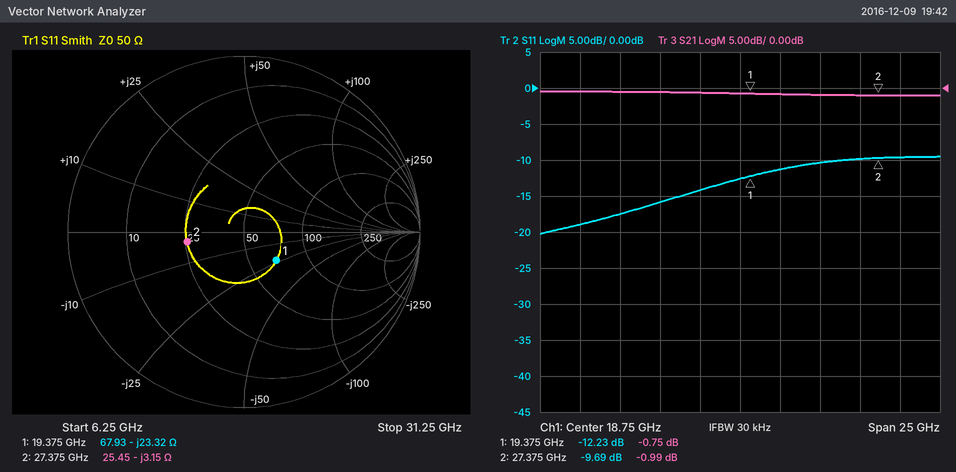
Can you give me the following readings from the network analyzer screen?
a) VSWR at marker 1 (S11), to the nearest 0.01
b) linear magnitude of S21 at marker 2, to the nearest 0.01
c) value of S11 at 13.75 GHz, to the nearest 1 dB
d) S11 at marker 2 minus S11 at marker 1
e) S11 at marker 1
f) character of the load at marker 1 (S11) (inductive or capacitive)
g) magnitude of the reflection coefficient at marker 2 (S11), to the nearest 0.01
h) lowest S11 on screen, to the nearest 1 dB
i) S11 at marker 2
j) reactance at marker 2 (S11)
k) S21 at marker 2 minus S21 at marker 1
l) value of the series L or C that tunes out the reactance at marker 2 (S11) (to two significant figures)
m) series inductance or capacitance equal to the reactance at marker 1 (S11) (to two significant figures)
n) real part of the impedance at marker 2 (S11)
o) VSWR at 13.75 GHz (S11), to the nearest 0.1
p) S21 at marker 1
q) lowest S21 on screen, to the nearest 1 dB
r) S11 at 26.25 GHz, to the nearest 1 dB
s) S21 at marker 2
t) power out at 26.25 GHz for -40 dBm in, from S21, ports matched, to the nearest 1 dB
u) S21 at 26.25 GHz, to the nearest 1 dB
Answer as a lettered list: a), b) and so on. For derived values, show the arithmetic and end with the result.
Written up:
a) (1 + 0.2446)/(1 − 0.2446) ≈ 1.65
b) 10^(-0.99/20) ≈ 0.89
c) -16 dB
d) -9.69 − (-12.23) = 2.54 dB
e) -12.23 dB
f) capacitive
g) 0.33
h) -20 dB
i) -9.69 dB
j) -3.15 Ω
k) -0.99 − (-0.75) = -0.24 dB
l) L = 3.15 Ω/(2π × 27.375 GHz) ≈ 18 pH
m) C = 1/(2π × 19.375 GHz × 23.32 Ω) ≈ 352 fF, so 350 fF to two significant figures
n) 25.45 Ω
o) |Γ| = 10^(-16/20) = 0.1585; VSWR = (1 + 0.1585)/(1 − 0.1585) ≈ 1.4
p) -0.75 dB
q) -1 dB
r) -10 dB
s) -0.99 dB
t) -40 dBm + (-1 dB) = -41 dBm
u) -1 dB
